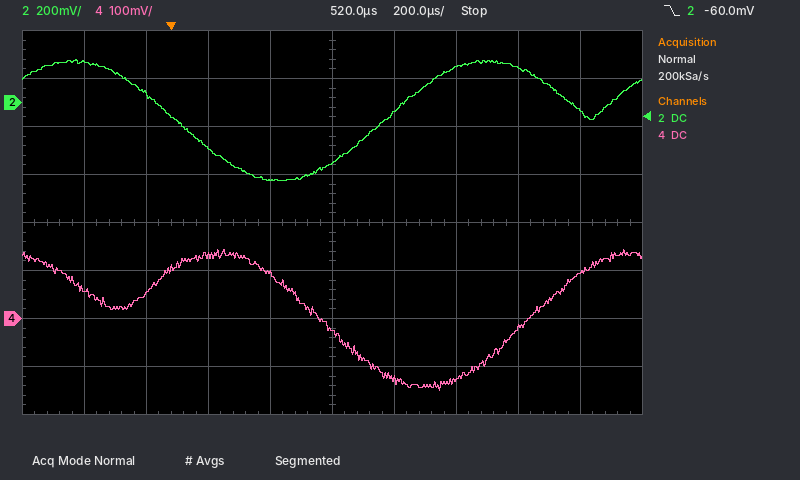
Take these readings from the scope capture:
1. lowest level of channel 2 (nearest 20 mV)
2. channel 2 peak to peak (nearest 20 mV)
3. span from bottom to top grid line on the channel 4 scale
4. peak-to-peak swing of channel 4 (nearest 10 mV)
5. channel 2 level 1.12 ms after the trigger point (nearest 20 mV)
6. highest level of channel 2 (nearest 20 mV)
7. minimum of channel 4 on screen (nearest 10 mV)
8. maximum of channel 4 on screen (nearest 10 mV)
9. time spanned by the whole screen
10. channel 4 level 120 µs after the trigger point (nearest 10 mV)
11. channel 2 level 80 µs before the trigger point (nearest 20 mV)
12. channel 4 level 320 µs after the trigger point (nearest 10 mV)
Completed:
-320 mV
500 mV
800 mV
290 mV
140 mV
180 mV
-150 mV
140 mV
2 ms
130 mV
40 mV
90 mV
